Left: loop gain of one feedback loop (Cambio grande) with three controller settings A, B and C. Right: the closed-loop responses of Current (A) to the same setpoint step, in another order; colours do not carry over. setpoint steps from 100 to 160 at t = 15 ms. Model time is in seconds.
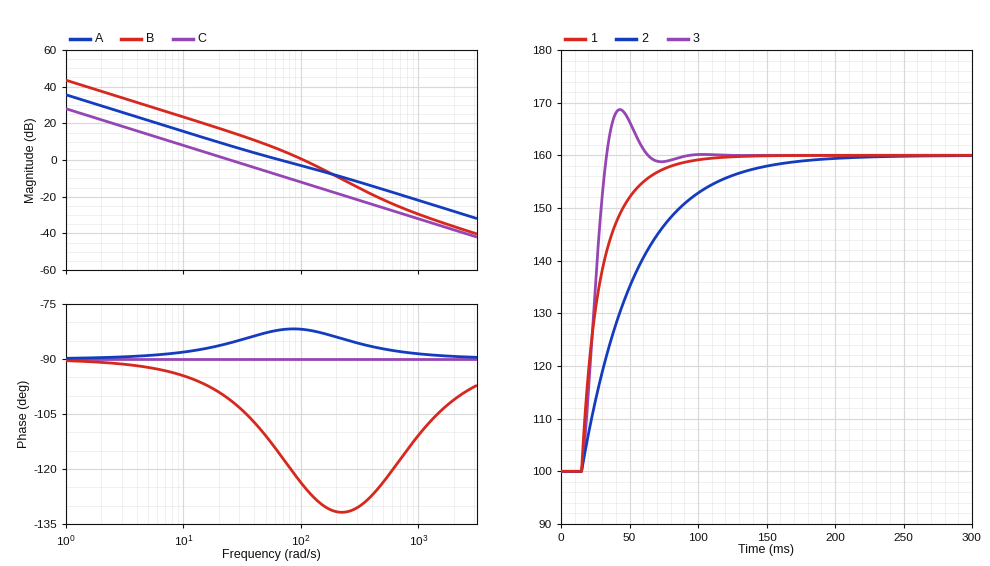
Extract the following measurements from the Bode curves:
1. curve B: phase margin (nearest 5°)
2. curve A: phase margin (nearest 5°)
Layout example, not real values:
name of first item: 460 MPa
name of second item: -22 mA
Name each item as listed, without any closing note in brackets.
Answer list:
curve B: phase margin: 55°
curve A: phase margin: 100°
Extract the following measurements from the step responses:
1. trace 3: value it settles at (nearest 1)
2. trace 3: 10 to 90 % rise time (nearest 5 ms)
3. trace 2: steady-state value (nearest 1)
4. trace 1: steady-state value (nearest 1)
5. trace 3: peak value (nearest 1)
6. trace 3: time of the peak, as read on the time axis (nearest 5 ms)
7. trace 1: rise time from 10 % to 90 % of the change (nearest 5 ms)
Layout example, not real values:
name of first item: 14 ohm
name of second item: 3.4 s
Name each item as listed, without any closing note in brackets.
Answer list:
trace 3: value it settles at: 160
trace 3: 10 to 90 % rise time: 15 ms
trace 2: steady-state value: 160
trace 1: steady-state value: 160
trace 3: peak value: 169
trace 3: time of the peak, as read on the time axis: 45 ms
trace 1: rise time from 10 % to 90 % of the change: 40 ms
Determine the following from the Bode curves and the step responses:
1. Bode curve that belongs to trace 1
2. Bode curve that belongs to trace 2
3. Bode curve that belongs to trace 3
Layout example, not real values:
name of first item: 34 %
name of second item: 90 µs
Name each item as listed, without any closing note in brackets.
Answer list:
Bode curve that belongs to trace 1: A
Bode curve that belongs to trace 2: C
Bode curve that belongs to trace 3: B
